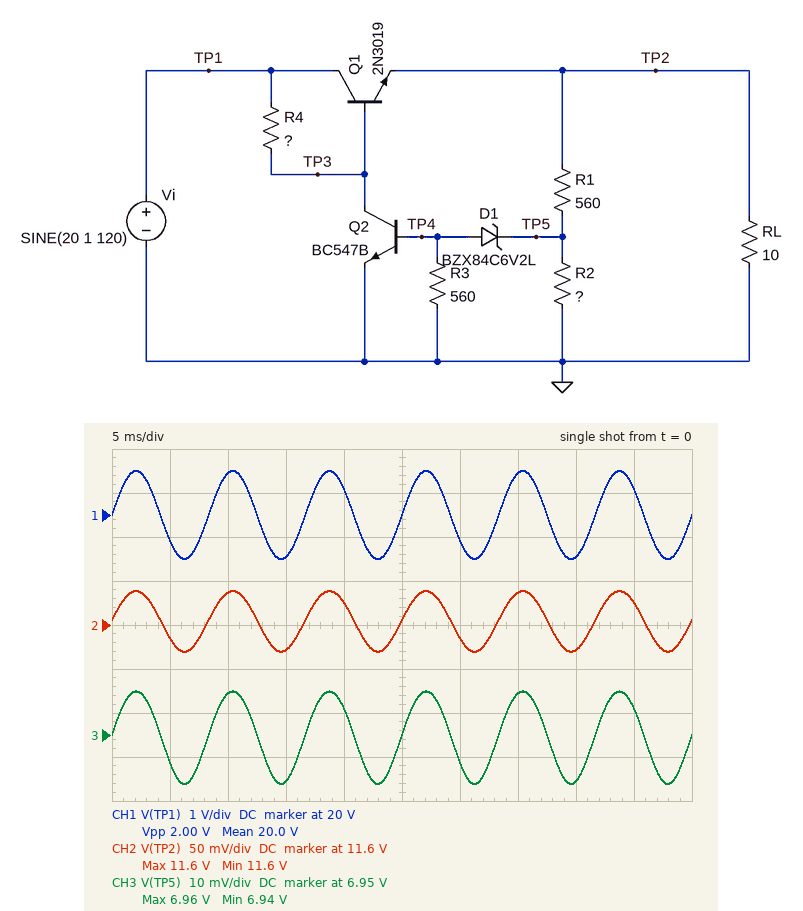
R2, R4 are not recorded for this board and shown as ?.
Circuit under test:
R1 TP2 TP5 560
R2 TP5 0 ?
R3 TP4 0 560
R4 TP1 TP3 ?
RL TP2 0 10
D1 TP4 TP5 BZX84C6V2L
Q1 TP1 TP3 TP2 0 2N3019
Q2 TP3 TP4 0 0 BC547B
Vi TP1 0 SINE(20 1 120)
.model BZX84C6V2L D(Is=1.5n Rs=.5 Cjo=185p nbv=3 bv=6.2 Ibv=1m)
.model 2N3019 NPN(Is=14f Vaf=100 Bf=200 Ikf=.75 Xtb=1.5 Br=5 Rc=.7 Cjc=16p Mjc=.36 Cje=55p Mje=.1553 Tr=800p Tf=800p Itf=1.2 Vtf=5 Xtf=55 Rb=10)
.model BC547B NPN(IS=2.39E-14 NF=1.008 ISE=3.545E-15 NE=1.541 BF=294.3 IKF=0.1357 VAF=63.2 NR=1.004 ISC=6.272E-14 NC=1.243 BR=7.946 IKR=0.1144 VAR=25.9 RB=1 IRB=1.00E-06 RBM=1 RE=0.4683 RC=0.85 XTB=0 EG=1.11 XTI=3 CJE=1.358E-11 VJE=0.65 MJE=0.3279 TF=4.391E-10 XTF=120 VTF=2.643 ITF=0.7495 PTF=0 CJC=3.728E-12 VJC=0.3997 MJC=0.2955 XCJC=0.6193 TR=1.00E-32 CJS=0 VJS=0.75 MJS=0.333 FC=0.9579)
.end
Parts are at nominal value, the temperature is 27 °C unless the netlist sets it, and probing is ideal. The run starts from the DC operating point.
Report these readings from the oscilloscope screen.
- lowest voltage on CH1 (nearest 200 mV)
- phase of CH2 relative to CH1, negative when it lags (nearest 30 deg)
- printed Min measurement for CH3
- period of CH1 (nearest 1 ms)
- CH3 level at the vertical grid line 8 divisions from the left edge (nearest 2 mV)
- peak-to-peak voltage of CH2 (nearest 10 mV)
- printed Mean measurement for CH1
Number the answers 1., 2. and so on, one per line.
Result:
1. 19.0 V
2. 0 deg
3. 6.94 V
4. 8 ms
5. 6.940 V
6. 70 mV
7. 20.0 V
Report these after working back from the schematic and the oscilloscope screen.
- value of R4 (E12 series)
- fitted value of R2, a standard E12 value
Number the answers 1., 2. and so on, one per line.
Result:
1. 220 Ω
2. 1 kΩ
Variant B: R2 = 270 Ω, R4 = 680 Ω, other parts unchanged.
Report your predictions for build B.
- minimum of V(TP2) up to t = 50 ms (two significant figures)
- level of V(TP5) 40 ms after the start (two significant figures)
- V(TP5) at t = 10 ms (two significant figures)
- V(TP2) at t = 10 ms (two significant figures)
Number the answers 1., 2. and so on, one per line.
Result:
1. 10 V
2. 3.4 V
3. 3.7 V
4. 11 V
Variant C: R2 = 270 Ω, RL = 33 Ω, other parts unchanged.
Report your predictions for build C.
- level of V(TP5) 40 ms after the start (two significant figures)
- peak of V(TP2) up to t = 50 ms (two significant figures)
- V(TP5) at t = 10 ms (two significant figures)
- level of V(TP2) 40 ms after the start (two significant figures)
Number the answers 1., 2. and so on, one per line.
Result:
1. 5.6 V
2. 19 V
3. 6.1 V
4. 17 V
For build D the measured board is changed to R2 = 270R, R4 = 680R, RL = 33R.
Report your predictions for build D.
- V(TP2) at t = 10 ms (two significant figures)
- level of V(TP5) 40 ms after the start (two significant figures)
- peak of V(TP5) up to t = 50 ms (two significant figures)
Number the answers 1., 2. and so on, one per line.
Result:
1. 17 V
2. 5.1 V
3. 5.6 V
